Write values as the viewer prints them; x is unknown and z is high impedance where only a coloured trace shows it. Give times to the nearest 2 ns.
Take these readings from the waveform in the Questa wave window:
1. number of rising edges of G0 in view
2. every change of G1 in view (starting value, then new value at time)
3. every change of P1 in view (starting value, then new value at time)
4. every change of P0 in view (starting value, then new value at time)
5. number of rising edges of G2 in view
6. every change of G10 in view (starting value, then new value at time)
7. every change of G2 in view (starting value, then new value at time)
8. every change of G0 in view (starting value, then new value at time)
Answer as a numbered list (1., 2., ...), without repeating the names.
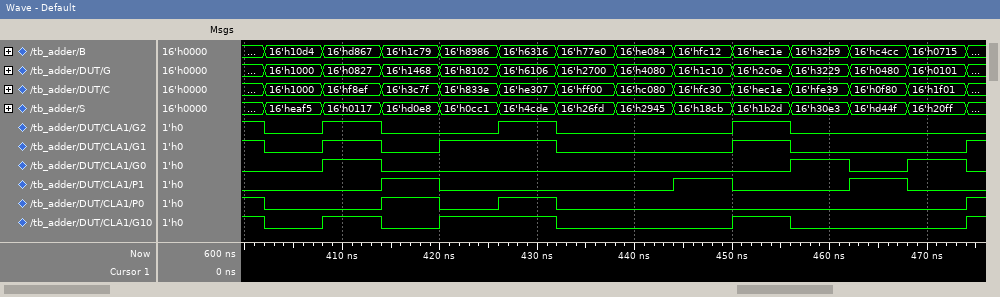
1. 3
2. 1, 0 at 402 ns, 1 at 408 ns, 0 at 414 ns, 1 at 420 ns, 0 at 432 ns, 1 at 450 ns, 0 at 456 ns, 1 at 474 ns
3. 0, 1 at 414 ns, 0 at 420 ns, 1 at 444 ns, 0 at 450 ns, 1 at 462 ns, 0 at 468 ns
4. 1, 0 at 402 ns, 1 at 414 ns, 0 at 420 ns, 1 at 426 ns, 0 at 432 ns, 1 at 474 ns
5. 3
6. 1, 0 at 402 ns, 1 at 408 ns, 0 at 414 ns, 1 at 420 ns, 0 at 432 ns, 1 at 450 ns, 0 at 456 ns, 1 at 474 ns
7. 1, 0 at 402 ns, 1 at 408 ns, 0 at 414 ns, 1 at 426 ns, 0 at 432 ns, 1 at 450 ns, 0 at 456 ns
8. 0, 1 at 408 ns, 0 at 414 ns, 1 at 456 ns, 0 at 462 ns, 1 at 468 ns, 0 at 474 ns
